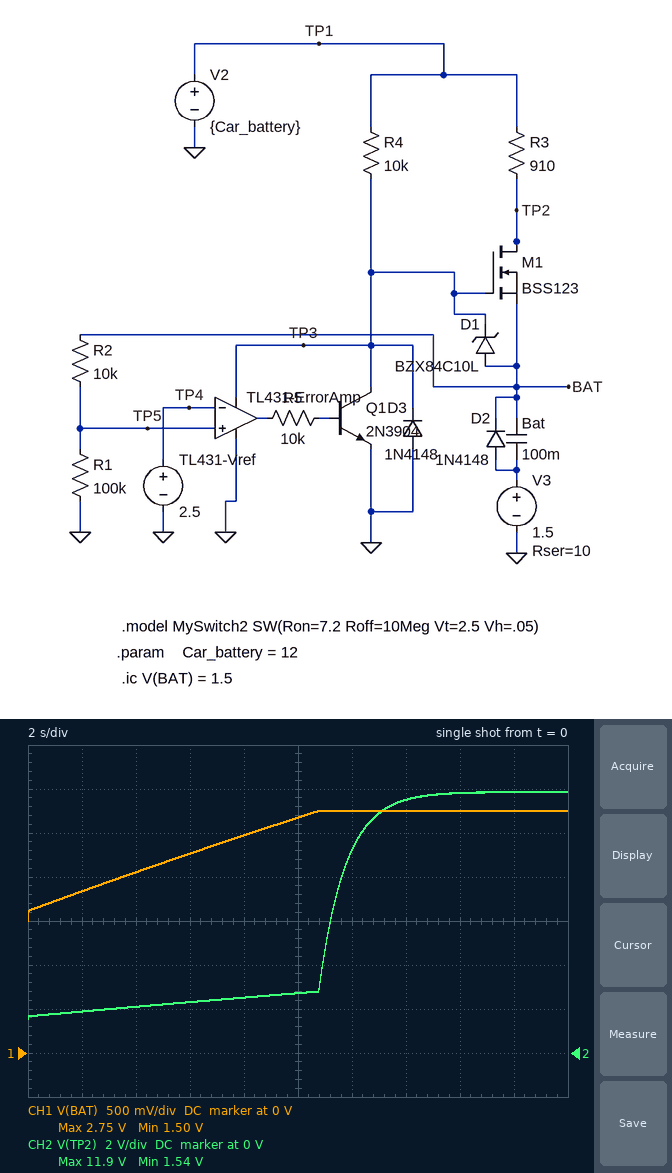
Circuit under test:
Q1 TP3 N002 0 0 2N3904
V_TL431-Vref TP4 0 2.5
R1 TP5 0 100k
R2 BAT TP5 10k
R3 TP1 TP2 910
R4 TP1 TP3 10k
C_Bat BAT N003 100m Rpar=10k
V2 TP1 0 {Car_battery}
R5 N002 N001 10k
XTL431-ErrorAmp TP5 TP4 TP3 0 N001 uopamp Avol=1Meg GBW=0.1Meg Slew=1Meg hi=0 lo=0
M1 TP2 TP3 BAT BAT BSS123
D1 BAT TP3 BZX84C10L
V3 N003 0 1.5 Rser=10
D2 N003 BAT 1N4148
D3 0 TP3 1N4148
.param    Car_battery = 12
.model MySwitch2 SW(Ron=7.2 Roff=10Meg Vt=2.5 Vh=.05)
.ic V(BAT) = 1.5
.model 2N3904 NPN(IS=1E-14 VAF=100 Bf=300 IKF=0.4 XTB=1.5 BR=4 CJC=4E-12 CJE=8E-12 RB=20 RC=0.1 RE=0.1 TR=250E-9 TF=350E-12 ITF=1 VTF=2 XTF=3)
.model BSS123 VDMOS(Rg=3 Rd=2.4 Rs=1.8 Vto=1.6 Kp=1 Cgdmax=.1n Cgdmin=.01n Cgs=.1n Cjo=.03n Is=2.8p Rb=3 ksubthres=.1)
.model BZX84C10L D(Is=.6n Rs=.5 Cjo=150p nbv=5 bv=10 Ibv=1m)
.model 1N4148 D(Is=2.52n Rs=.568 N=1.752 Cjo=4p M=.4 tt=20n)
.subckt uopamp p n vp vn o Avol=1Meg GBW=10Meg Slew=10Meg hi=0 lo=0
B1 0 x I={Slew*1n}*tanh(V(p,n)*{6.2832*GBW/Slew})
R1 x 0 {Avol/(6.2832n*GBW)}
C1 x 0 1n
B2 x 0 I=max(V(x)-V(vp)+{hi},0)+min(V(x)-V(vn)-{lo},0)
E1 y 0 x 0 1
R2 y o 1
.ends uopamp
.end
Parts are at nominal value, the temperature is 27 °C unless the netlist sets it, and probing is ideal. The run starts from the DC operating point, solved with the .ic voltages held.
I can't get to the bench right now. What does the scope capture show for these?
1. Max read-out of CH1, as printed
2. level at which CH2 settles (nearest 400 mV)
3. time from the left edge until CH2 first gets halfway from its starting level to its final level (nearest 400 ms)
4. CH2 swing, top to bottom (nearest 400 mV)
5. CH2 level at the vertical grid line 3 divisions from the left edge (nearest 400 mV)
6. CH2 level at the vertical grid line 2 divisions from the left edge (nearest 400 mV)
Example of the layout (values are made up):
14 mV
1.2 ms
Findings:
2.75 V
12.0 V
11.2 s
10.4 V
2.4 V
2.0 V
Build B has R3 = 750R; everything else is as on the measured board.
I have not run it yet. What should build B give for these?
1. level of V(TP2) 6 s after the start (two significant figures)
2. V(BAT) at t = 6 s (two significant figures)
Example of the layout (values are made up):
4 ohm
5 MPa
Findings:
2.5 V
2.4 V
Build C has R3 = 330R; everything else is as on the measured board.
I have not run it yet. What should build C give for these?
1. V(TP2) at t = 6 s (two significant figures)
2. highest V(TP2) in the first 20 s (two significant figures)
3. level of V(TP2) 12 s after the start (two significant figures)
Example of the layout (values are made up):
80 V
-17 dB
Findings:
11 V
12 V
12 V
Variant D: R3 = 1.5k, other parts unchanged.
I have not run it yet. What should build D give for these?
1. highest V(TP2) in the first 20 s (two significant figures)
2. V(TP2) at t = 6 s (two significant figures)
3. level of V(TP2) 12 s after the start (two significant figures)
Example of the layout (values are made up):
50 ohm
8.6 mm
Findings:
10 V
2.0 V
2.4 V
